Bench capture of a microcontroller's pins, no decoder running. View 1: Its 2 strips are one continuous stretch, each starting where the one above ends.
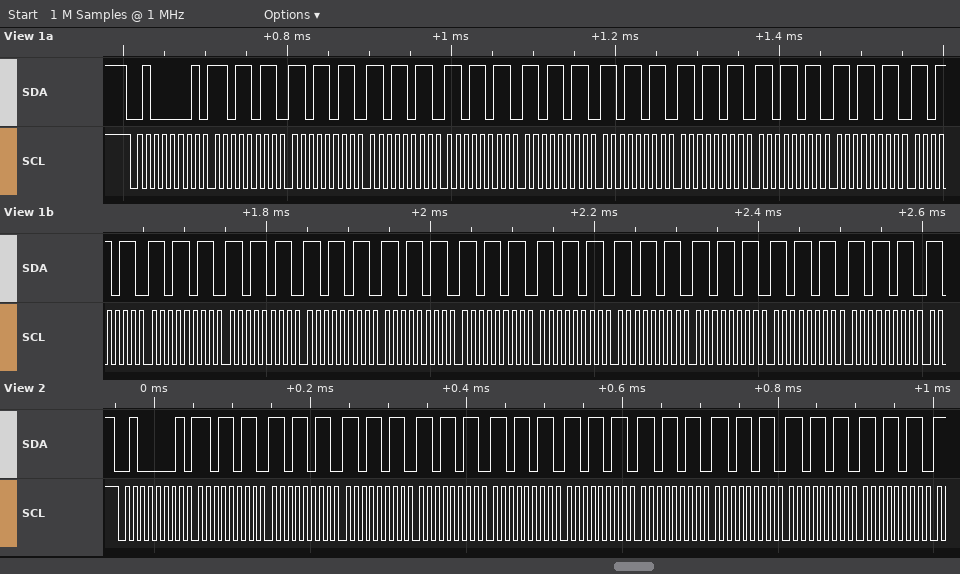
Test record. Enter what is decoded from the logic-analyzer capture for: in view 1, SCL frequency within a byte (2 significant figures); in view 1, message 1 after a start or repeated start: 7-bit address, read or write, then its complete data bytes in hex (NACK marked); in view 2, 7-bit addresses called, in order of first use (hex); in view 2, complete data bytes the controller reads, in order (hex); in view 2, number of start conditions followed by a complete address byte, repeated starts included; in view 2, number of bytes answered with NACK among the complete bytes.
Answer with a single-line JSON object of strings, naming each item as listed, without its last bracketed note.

{"in view 1, SCL frequency within a byte": "100 kHz", "in view 1, message 1 after a start or repeated start: 7-bit address, read or write, then its complete data bytes in hex": "0x20 read: DB DB DB DB DB DB DB DB DB DB DB DB DB DB DB DB DB DB DB DB", "in view 2, 7-bit addresses called, in order of first use": "0x20", "in view 2, complete data bytes the controller reads, in order": "DB DB DB DB DB DB DB DB DB DB", "in view 2, number of start conditions followed by a complete address byte, repeated starts included": "1", "in view 2, number of bytes answered with NACK among the complete bytes": "0"}
